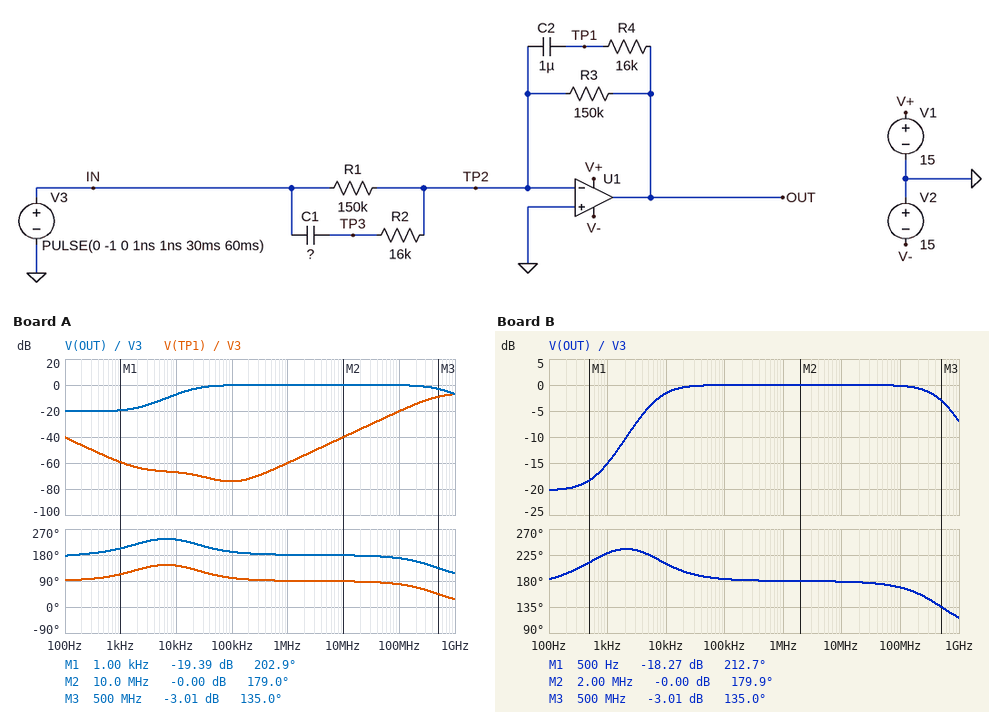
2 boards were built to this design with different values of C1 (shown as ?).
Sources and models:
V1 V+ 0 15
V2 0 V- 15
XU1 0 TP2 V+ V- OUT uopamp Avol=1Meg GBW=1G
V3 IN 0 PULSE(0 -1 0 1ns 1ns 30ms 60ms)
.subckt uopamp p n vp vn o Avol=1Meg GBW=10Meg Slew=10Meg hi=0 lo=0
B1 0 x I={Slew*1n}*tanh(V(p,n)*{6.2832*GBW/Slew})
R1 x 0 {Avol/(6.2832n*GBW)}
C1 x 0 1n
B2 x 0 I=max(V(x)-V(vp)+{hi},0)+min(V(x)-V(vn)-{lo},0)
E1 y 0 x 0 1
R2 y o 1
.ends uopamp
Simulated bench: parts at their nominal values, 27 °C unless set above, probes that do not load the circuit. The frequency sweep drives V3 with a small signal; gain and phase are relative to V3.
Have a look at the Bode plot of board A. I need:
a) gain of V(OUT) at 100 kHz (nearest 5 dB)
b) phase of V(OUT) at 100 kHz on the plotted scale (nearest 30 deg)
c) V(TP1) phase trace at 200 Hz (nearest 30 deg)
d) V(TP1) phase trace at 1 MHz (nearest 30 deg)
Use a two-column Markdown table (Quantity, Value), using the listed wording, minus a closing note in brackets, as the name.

| Quantity | Value |
|---|---|
| gain of V(OUT) at 100 kHz | 0 dB |
| phase of V(OUT) at 100 kHz on the plotted scale | 180 deg |
| V(TP1) phase trace at 200 Hz | 90 deg |
| V(TP1) phase trace at 1 MHz | 90 deg |
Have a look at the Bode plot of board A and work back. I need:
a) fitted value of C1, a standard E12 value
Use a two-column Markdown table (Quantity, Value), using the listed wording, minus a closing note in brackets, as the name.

| Quantity | Value |
|---|---|
| fitted value of C1, a standard E12 value | 470 pF |
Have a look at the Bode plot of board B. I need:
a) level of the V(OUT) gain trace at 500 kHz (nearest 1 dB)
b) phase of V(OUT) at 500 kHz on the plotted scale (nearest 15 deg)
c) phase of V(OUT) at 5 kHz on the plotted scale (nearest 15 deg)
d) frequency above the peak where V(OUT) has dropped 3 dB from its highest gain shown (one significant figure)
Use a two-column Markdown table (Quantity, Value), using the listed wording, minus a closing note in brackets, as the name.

| Quantity | Value |
|---|---|
| level of the V(OUT) gain trace at 500 kHz | 0 dB |
| phase of V(OUT) at 500 kHz on the plotted scale | 180 deg |
| phase of V(OUT) at 5 kHz on the plotted scale | 225 deg |
| frequency above the peak where V(OUT) has dropped 3 dB from its highest gain shown | 500 MHz |
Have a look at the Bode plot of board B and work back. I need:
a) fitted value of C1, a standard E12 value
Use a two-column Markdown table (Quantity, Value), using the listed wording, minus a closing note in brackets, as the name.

| Quantity | Value |
|---|---|
| fitted value of C1, a standard E12 value | 1.5 nF |
